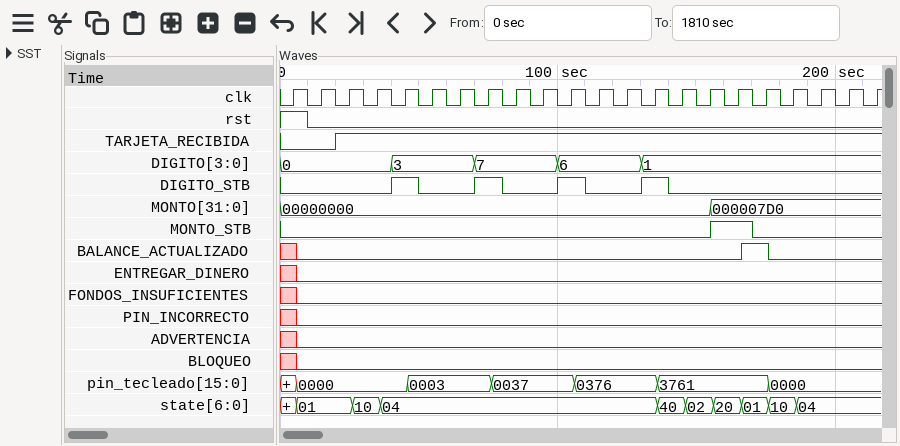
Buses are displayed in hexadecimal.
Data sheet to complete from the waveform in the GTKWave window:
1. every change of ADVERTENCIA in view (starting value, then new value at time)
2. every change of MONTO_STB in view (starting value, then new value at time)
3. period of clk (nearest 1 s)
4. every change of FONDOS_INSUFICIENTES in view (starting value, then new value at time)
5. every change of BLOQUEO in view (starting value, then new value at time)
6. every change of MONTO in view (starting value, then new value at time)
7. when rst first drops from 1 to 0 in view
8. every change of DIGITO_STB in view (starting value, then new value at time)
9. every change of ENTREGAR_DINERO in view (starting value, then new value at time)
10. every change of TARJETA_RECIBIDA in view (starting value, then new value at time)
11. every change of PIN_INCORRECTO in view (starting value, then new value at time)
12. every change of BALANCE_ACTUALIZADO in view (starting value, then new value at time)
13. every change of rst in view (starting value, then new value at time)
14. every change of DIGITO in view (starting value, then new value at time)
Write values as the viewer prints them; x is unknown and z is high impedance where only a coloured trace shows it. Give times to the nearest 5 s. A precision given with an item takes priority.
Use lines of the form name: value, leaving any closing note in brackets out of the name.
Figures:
every change of ADVERTENCIA in view: x, 0 at 5 s
every change of MONTO_STB in view: 0, 1 at 155 s, 0 at 170 s
period of clk: 10 s
every change of FONDOS_INSUFICIENTES in view: x, 0 at 5 s
every change of BLOQUEO in view: x, 0 at 5 s
every change of MONTO in view: 00000000, 000007D0 at 155 s
when rst first drops from 1 to 0 in view: 10 s
every change of DIGITO_STB in view: 0, 1 at 40 s, 0 at 50 s, 1 at 70 s, 0 at 80 s, 1 at 100 s, 0 at 110 s, 1 at 130 s, 0 at 140 s
every change of ENTREGAR_DINERO in view: x, 0 at 5 s
every change of TARJETA_RECIBIDA in view: 0, 1 at 20 s
every change of PIN_INCORRECTO in view: x, 0 at 5 s
every change of BALANCE_ACTUALIZADO in view: x, 0 at 5 s, 1 at 165 s, 0 at 175 s
every change of rst in view: 1, 0 at 10 s
every change of DIGITO in view: 0, 3 at 40 s, 7 at 70 s, 6 at 100 s, 1 at 130 s
